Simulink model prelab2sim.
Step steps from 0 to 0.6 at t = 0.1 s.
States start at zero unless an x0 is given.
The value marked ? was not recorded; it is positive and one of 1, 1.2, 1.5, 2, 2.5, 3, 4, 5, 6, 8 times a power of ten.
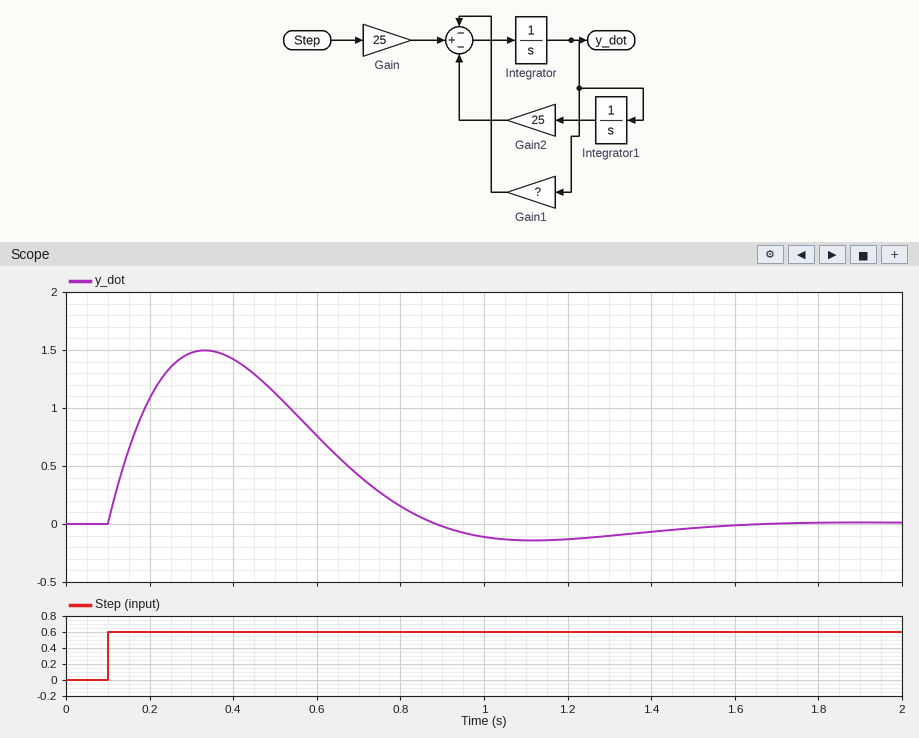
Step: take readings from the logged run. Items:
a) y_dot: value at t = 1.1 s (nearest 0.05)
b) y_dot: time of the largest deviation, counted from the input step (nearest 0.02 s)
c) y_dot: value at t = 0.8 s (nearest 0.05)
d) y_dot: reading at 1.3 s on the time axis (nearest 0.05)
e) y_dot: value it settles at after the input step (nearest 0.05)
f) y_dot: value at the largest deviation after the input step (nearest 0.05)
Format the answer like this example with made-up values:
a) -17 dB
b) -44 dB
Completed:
a) -0.15
b) 0.24 s
c) 0.15
d) -0.10
e) 0.00
f) 1.50
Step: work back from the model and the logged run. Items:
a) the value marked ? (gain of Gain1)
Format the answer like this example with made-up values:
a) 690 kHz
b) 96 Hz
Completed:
a) 6
